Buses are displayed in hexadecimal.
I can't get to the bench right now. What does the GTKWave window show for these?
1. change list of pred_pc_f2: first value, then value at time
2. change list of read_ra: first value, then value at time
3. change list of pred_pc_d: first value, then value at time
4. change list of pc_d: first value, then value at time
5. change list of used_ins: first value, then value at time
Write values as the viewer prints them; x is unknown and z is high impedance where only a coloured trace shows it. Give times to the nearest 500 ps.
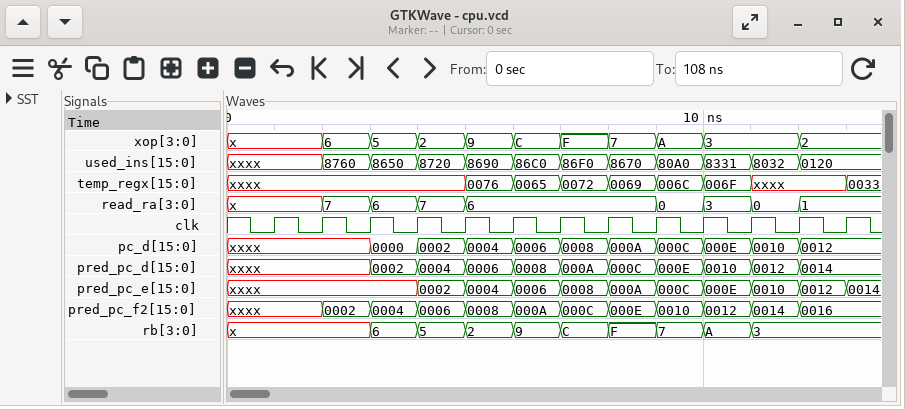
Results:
xxxx, 0002 at 2000 ps, 0004 at 3000 ps, 0006 at 4000 ps, 0008 at 5000 ps, 000A at 6000 ps, 000C at 7000 ps, 000E at 8000 ps, 0010 at 9000 ps, 0012 at 10000 ps, 0014 at 11000 ps, 0016 at 12000 ps
x, 7 at 2000 ps, 6 at 3000 ps, 7 at 4000 ps, 6 at 5000 ps, 0 at 9000 ps, 3 at 10000 ps, 0 at 11000 ps, 1 at 12000 ps
xxxx, 0002 at 3000 ps, 0004 at 4000 ps, 0006 at 5000 ps, 0008 at 6000 ps, 000A at 7000 ps, 000C at 8000 ps, 000E at 9000 ps, 0010 at 10000 ps, 0012 at 11000 ps, 0014 at 12000 ps
xxxx, 0000 at 3000 ps, 0002 at 4000 ps, 0004 at 5000 ps, 0006 at 6000 ps, 0008 at 7000 ps, 000A at 8000 ps, 000C at 9000 ps, 000E at 10000 ps, 0010 at 11000 ps, 0012 at 12000 ps
xxxx, 8760 at 2000 ps, 8650 at 3000 ps, 8720 at 4000 ps, 8690 at 5000 ps, 86C0 at 6000 ps, 86F0 at 7000 ps, 8670 at 8000 ps, 80A0 at 9000 ps, 8331 at 10000 ps, 8032 at 11000 ps, 0120 at 12000 ps
